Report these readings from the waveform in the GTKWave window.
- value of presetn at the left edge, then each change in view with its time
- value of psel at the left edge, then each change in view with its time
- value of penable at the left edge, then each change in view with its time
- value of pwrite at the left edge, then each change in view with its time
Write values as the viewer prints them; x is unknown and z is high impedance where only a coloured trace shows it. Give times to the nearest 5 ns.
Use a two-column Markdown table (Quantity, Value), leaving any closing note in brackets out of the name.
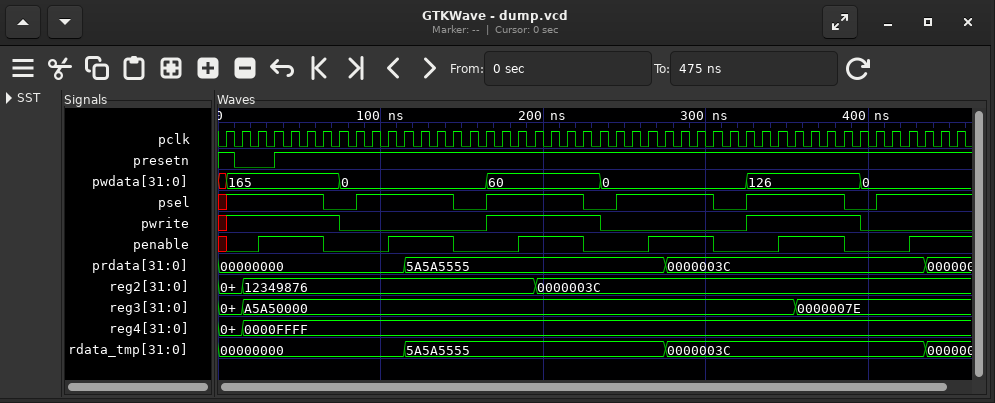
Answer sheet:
| Quantity | Value |
|---|---|
| value of presetn at the left edge, then each change in view with its time | 1, 0 at 10 ns, 1 at 35 ns |
| value of psel at the left edge, then each change in view with its time | x, 1 at 5 ns, 0 at 65 ns, 1 at 85 ns, 0 at 145 ns, 1 at 165 ns, 0 at 225 ns, 1 at 245 ns, 0 at 305 ns, 1 at 325 ns, 0 at 385 ns, 1 at 405 ns |
| value of penable at the left edge, then each change in view with its time | x, 0 at 5 ns, 1 at 25 ns, 0 at 65 ns, 1 at 105 ns, 0 at 145 ns, 1 at 185 ns, 0 at 225 ns, 1 at 265 ns, 0 at 305 ns, 1 at 345 ns, 0 at 385 ns, 1 at 425 ns |
| value of pwrite at the left edge, then each change in view with its time | x, 1 at 5 ns, 0 at 75 ns, 1 at 165 ns, 0 at 235 ns, 1 at 325 ns, 0 at 395 ns |
